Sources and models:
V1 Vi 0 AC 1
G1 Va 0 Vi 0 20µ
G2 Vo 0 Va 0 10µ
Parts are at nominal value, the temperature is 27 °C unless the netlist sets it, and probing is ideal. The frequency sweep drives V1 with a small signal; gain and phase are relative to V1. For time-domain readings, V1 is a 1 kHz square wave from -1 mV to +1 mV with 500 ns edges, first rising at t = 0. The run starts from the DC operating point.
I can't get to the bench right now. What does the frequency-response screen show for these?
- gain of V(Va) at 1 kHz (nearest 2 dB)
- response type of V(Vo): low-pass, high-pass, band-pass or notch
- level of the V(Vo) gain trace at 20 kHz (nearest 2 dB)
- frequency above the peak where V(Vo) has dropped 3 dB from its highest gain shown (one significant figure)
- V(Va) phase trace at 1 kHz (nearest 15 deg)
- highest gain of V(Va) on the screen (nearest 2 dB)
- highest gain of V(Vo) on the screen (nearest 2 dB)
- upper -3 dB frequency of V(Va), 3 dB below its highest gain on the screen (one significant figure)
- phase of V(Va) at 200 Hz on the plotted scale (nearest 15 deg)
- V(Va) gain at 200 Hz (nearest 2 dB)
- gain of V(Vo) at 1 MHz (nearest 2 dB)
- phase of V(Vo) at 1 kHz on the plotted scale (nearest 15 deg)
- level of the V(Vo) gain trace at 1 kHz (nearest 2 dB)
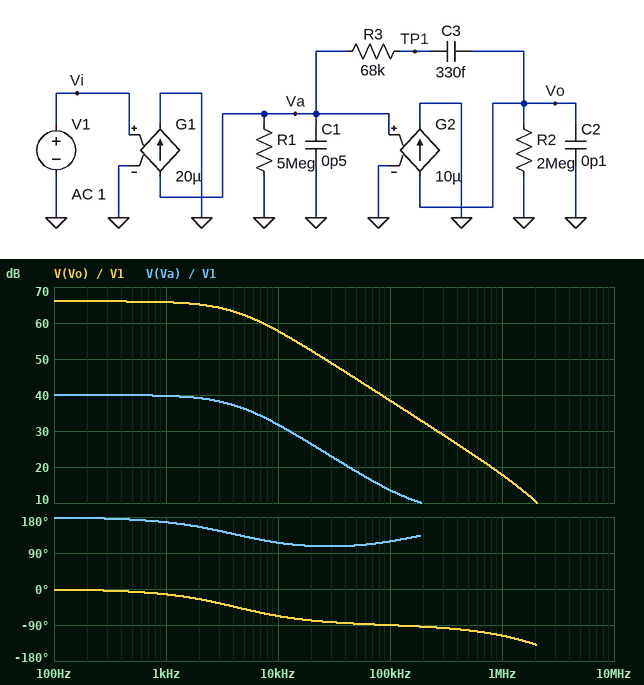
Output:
40 dB
low-pass
52 dB
4 kHz
165 deg
40 dB
66 dB
4 kHz
180 deg
40 dB
18 dB
-15 deg
66 dB
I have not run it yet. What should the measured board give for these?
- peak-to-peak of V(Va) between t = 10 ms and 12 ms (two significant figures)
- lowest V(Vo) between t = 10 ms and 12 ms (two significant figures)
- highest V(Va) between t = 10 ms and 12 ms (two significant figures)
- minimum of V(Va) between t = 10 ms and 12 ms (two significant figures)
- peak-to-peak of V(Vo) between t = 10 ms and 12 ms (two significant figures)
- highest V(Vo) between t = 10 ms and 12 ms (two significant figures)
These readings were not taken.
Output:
200 mV
-2.0 V
100 mV
-100 mV
4.0 V
2.0 V
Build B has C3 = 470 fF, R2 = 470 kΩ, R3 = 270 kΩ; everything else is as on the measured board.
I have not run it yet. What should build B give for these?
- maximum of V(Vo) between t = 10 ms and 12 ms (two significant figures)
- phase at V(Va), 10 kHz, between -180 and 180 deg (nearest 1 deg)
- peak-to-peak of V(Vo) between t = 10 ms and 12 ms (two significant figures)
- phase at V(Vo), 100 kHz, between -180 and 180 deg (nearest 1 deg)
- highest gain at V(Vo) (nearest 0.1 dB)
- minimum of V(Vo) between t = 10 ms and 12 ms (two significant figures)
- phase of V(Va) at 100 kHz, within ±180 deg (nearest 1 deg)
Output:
470 mV
136 deg
940 mV
-84 deg
53.4 dB
-470 mV
107 deg
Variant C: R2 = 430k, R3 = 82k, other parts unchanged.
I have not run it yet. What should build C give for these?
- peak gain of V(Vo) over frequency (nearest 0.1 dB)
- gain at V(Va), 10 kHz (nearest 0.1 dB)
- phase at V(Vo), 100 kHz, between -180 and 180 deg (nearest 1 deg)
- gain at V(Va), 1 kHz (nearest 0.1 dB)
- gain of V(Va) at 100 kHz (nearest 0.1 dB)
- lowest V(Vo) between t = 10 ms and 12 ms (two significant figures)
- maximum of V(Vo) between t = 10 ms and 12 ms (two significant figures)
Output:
52.7 dB
38.2 dB
-84 deg
40.0 dB
22.9 dB
-430 mV
430 mV
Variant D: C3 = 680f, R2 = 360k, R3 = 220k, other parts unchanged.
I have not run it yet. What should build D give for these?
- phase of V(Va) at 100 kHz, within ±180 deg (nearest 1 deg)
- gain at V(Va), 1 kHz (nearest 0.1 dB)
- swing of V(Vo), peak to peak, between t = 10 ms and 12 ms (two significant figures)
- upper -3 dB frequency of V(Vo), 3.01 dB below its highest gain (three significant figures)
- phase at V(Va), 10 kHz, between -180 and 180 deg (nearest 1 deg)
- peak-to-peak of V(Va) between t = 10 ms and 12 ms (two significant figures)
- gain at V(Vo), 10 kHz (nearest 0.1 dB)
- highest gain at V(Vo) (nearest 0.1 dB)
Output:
108 deg
39.9 dB
720 mV
8.60 kHz
132 deg
200 mV
47.4 dB
51.1 dB
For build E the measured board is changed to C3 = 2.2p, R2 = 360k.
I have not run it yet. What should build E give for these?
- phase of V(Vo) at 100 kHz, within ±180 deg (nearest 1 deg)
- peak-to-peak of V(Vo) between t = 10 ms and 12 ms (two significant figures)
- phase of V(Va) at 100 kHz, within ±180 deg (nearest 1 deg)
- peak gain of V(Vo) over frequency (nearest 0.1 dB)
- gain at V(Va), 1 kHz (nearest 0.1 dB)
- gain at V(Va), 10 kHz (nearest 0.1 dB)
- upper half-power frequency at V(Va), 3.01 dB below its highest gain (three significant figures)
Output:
-93 deg
720 mV
121 deg
51.1 dB
39.5 dB
29.0 dB
2.95 kHz
